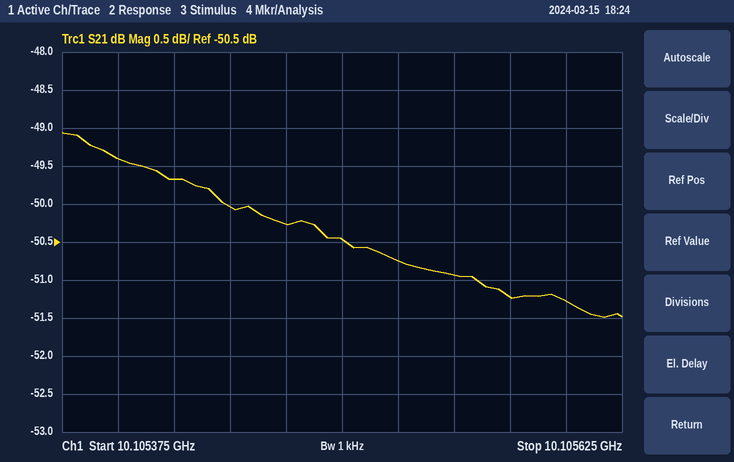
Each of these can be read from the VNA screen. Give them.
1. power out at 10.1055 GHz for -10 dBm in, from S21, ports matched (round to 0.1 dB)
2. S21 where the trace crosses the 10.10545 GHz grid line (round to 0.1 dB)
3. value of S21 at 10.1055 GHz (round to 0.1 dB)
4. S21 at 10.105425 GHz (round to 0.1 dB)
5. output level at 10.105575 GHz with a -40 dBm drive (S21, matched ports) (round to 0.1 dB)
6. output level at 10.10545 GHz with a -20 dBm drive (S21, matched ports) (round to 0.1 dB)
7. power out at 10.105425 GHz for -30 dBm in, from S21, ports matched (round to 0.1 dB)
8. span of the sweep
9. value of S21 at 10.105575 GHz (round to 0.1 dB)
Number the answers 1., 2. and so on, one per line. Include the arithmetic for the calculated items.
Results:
1. -10 dBm + (-50.5 dB) = -60.5 dBm
2. -50.0 dB
3. -50.5 dB
4. -49.7 dB
5. -40 dBm + (-51.2 dB) = -91.2 dBm
6. -20 dBm + (-50.0 dB) = -70.0 dBm
7. -30 dBm + (-49.7 dB) = -79.7 dBm
8. 250 kHz
9. -51.2 dB
